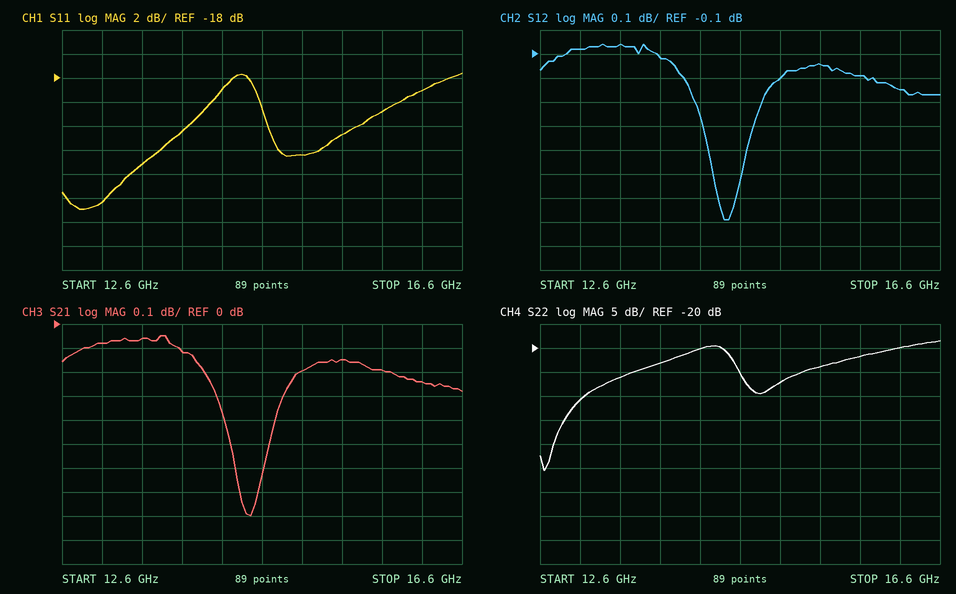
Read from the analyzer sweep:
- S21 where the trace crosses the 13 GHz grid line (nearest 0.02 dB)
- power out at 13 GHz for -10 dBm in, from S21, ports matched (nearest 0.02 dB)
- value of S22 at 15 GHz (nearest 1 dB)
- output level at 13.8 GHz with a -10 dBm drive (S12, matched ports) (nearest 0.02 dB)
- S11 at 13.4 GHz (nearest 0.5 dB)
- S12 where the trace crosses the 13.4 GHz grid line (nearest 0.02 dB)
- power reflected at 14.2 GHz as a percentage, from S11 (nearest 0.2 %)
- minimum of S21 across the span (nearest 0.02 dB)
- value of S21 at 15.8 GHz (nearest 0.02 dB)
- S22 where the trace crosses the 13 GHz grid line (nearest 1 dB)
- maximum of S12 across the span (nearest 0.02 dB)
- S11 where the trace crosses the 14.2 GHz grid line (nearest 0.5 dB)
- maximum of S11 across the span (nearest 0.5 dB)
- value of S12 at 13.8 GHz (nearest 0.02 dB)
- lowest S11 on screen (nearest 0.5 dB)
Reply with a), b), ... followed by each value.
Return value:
a) -0.08 dB
b) -10.08 dBm
c) -27 dB
d) -10.12 dBm
e) -25.0 dB
f) -0.06 dB
g) 1.2 %
h) -0.80 dB
i) -0.20 dB
j) -31 dB
k) -0.06 dB
l) -19.0 dB
m) -17.5 dB
n) -0.12 dB
o) -29.0 dB
